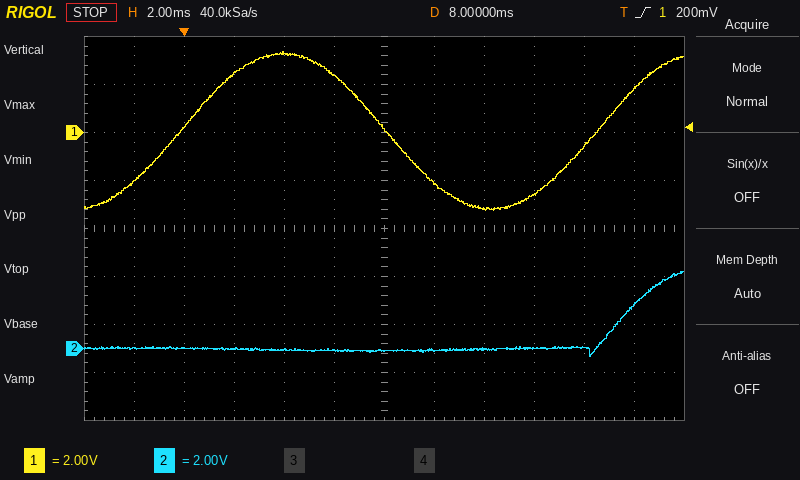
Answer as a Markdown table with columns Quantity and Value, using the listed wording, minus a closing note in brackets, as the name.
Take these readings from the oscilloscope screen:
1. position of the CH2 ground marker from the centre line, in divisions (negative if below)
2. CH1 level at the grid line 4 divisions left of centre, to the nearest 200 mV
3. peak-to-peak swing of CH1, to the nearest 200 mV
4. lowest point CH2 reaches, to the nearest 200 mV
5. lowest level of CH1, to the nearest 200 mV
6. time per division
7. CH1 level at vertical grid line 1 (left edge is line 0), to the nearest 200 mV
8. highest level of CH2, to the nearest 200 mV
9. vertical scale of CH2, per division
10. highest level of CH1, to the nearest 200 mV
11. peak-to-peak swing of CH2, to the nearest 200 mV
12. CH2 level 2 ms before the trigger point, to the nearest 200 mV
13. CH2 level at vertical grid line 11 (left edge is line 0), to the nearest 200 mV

| Quantity | Value |
|---|---|
| position of the CH2 ground marker from the centre line, in divisions | -2.5 div |
| CH1 level at the grid line 4 divisions left of centre, to the nearest 200 mV | 200 mV |
| peak-to-peak swing of CH1, to the nearest 200 mV | 6.6 V |
| lowest point CH2 reaches, to the nearest 200 mV | -400 mV |
| lowest level of CH1, to the nearest 200 mV | -3.2 V |
| time per division | 2 ms |
| CH1 level at vertical grid line 1 (left edge is line 0), to the nearest 200 mV | -2.0 V |
| highest level of CH2, to the nearest 200 mV | 3.2 V |
| vertical scale of CH2, per division | 2 V |
| highest level of CH1, to the nearest 200 mV | 3.4 V |
| peak-to-peak swing of CH2, to the nearest 200 mV | 3.6 V |
| CH2 level 2 ms before the trigger point, to the nearest 200 mV | 0.0 V |
| CH2 level at vertical grid line 11 (left edge is line 0), to the nearest 200 mV | 1.8 V |
